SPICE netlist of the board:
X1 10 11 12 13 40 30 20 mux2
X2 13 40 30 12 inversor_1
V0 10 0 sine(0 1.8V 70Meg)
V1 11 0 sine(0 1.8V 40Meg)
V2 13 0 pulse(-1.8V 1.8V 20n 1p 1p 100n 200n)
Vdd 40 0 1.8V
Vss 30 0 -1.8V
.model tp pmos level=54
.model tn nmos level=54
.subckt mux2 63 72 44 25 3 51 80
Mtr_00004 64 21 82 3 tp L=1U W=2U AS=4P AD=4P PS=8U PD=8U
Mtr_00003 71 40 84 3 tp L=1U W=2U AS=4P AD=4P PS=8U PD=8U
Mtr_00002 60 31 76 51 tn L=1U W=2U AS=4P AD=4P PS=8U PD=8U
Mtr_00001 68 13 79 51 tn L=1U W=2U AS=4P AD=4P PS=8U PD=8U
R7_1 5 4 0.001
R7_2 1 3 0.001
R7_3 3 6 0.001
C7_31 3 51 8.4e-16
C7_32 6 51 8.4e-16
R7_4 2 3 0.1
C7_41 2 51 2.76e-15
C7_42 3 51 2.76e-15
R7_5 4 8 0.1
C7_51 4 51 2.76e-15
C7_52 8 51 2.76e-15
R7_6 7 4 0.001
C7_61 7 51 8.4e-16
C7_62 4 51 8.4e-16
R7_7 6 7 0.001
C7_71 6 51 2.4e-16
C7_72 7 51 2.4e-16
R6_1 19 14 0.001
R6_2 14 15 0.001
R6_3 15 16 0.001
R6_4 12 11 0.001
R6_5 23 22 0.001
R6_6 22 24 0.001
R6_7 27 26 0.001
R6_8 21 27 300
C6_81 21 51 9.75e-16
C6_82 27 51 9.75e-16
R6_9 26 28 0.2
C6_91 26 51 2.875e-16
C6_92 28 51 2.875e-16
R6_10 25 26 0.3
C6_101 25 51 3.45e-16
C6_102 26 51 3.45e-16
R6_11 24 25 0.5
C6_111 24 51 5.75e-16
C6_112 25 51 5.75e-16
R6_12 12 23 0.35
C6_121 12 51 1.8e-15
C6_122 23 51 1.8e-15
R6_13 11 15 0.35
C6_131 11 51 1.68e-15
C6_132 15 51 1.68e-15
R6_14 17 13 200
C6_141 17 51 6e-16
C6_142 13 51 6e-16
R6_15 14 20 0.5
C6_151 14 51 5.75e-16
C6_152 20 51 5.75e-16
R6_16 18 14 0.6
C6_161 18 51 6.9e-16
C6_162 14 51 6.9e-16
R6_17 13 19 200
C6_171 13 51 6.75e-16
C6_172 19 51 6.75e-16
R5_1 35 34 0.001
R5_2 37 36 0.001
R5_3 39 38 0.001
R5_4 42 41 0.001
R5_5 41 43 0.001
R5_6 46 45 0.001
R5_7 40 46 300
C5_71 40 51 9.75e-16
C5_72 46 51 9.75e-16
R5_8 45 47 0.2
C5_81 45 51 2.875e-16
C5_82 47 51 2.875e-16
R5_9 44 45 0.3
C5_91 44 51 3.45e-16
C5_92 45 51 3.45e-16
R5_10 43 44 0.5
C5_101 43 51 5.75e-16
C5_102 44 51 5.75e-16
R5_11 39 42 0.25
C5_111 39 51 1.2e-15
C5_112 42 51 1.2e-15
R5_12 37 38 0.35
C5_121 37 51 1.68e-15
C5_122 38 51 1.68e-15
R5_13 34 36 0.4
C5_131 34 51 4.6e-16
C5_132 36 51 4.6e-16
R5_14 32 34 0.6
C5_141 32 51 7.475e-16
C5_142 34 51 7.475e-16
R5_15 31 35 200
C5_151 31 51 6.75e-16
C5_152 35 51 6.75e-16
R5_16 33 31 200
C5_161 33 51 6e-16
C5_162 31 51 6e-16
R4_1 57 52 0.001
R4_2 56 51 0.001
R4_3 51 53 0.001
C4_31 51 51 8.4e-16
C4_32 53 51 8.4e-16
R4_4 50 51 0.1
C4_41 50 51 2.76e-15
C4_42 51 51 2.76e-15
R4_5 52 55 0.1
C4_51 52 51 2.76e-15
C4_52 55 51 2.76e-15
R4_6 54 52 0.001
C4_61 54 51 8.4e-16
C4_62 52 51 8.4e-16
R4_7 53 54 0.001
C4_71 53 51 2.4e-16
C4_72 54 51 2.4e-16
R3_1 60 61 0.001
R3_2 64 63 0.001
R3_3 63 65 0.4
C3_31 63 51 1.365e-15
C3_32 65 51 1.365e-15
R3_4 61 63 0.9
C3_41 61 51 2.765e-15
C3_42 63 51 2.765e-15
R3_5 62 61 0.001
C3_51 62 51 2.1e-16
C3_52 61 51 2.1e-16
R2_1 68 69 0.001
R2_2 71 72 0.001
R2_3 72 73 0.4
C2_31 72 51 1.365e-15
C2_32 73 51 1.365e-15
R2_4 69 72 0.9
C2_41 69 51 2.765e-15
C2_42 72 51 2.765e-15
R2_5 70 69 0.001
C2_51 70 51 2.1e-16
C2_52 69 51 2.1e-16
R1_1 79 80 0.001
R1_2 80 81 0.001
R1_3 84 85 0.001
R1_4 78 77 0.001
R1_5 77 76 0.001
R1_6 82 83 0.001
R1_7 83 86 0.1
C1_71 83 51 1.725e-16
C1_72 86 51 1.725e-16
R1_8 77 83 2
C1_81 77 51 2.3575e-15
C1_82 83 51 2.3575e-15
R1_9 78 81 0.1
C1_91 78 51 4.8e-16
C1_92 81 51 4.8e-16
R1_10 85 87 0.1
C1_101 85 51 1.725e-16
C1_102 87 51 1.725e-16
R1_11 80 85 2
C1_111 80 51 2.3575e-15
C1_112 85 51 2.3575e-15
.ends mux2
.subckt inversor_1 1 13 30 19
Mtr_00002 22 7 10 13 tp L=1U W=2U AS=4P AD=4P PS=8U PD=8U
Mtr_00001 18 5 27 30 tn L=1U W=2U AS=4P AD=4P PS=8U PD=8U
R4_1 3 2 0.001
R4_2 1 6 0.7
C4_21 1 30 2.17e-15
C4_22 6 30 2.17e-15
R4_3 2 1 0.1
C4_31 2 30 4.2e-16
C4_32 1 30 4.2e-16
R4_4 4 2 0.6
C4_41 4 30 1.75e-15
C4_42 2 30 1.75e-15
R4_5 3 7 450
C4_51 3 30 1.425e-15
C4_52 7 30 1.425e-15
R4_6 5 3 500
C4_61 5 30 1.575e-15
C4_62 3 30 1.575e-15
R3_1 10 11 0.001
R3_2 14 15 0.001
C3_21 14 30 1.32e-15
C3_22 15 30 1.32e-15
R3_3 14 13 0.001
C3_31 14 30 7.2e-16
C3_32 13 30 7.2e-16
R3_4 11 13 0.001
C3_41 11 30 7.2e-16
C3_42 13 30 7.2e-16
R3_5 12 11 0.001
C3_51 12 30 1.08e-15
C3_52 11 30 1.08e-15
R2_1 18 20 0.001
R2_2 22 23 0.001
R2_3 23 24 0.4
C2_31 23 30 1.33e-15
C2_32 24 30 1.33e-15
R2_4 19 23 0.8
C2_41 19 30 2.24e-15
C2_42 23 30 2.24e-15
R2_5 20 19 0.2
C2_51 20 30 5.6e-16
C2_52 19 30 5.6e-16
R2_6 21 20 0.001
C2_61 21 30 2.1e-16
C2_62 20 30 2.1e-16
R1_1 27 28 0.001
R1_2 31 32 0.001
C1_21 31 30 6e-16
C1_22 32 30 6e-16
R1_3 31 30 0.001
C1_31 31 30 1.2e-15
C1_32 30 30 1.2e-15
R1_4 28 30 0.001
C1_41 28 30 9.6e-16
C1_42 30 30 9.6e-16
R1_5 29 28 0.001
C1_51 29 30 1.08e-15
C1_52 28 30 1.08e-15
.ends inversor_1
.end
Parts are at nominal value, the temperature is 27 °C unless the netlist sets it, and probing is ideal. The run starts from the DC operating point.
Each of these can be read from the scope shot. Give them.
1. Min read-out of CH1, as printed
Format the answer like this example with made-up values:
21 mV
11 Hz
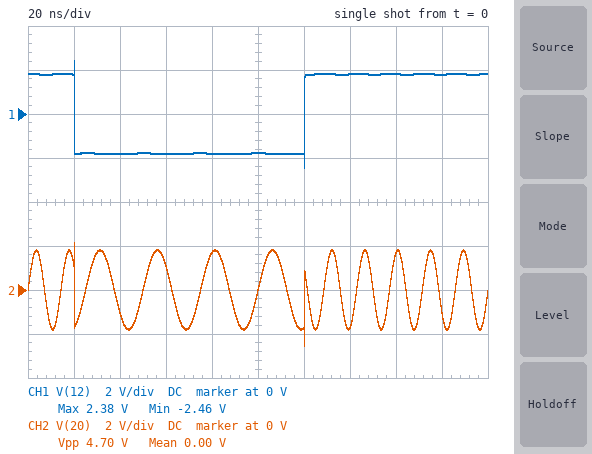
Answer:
-2.46 V
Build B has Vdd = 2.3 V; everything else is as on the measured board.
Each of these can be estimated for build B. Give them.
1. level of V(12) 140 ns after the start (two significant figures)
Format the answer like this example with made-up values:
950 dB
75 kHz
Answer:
2.3 V
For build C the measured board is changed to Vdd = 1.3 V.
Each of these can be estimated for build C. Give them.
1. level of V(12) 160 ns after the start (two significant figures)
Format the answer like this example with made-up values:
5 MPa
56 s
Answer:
1.3 V
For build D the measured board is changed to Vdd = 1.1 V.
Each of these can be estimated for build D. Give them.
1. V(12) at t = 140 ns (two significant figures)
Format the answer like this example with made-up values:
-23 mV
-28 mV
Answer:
1.1 V
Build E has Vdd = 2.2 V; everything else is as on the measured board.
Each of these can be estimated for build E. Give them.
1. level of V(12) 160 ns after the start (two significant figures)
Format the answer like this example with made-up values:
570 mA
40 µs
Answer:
2.2 V
